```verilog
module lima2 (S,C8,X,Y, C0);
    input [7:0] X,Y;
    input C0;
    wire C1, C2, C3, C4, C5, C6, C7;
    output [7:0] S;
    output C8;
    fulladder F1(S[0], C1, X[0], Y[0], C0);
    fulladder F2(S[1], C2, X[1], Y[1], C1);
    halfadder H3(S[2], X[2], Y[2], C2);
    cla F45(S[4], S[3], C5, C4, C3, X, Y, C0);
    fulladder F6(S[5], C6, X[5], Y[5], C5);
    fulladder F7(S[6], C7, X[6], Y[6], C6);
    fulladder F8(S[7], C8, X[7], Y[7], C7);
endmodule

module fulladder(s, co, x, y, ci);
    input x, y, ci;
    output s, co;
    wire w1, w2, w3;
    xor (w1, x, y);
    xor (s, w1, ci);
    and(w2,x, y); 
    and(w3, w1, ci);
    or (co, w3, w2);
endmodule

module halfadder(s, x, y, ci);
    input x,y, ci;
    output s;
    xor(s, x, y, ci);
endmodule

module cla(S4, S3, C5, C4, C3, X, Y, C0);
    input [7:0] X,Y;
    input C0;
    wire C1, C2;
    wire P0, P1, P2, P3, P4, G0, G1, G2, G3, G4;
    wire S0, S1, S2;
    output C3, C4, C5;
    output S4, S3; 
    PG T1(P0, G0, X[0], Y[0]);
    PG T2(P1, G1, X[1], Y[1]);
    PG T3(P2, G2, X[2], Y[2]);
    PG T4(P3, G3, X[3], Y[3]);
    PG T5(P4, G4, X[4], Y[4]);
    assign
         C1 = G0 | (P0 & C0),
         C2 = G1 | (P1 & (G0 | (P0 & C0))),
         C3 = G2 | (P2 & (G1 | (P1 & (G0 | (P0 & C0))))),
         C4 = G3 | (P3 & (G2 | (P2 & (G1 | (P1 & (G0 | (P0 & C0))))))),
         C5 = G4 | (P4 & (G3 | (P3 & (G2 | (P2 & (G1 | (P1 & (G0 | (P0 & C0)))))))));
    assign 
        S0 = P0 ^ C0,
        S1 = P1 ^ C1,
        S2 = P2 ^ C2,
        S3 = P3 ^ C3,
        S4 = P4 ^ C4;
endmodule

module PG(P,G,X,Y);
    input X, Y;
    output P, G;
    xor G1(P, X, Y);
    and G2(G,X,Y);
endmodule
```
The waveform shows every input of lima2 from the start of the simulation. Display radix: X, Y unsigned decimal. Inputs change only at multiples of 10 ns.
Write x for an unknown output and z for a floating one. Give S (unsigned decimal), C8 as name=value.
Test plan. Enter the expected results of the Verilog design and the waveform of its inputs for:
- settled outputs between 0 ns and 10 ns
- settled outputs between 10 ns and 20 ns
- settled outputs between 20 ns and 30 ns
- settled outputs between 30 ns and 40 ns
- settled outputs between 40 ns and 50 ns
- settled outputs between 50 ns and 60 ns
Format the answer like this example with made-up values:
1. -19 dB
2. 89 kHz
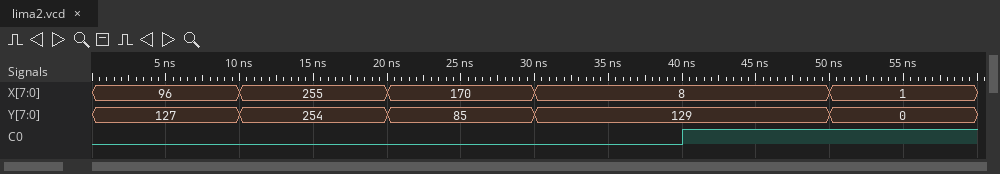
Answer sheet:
1. S=223, C8=0
2. S=253, C8=1
3. S=255, C8=0
4. S=137, C8=0
5. S=138, C8=0
6. S=2, C8=0
